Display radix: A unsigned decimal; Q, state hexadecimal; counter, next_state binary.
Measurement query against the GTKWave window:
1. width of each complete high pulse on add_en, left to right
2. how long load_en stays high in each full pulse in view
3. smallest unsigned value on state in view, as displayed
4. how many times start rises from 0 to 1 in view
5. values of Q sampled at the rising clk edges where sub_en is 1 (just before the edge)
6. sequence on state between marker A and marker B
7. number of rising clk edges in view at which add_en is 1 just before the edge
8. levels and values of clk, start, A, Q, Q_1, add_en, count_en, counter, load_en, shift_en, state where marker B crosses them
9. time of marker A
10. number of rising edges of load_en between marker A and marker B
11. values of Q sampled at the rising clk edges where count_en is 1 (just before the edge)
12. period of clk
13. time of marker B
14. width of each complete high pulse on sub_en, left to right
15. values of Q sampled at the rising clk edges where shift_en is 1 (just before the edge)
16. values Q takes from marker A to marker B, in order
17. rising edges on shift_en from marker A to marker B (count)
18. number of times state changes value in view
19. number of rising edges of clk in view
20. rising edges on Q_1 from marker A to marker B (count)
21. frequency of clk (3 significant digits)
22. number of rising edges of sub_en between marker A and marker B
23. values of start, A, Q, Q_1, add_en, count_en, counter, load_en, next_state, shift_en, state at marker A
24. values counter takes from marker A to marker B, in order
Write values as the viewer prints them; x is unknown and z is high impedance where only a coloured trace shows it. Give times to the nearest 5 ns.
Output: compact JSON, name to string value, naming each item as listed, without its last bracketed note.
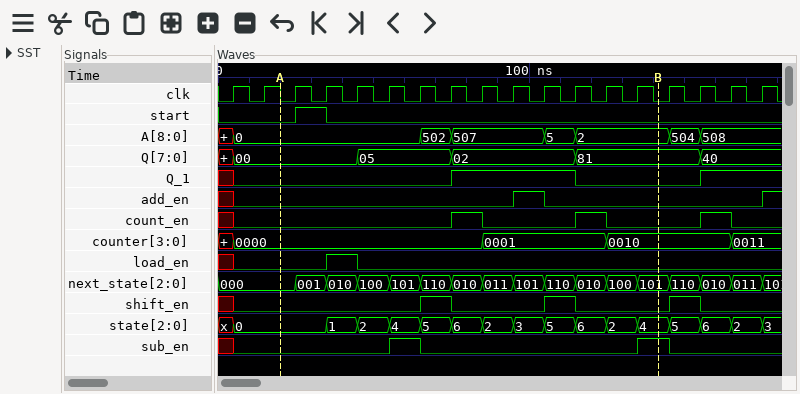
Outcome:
{"width of each complete high pulse on add_en, left to right": "10 ns", "how long load_en stays high in each full pulse in view": "10 ns", "smallest unsigned value on state in view, as displayed": "0", "how many times start rises from 0 to 1 in view": "1", "values of Q sampled at the rising clk edges where sub_en is 1": "05, 81", "sequence on state between marker A and marker B": "0, 1, 2, 4, 5, 6, 2, 3, 5, 6, 2, 4", "number of rising clk edges in view at which add_en is 1 just before the edge": "1", "levels and values of clk, start, A, Q, Q_1, add_en, count_en, counter, load_en, shift_en, state where marker B crosses them": "clk=0, start=0, A=2, Q=81, Q_1=0, add_en=0, count_en=0, counter=0010, load_en=0, shift_en=0, state=4", "time of marker A": "20 ns", "number of rising edges of load_en between marker A and marker B": "1", "values of Q sampled at the rising clk edges where count_en is 1": "02, 81, 40", "period of clk": "10 ns", "time of marker B": "140 ns", "width of each complete high pulse on sub_en, left to right": "10 ns, 10 ns", "values of Q sampled at the rising clk edges where shift_en is 1": "05, 02, 81", "values Q takes from marker A to marker B, in order": "00, 05, 02, 81", "rising edges on shift_en from marker A to marker B": "2", "number of times state changes value in view": "16", "number of rising edges of clk in view": "18", "rising edges on Q_1 from marker A to marker B": "1", "frequency of clk": "100 MHz", "number of rising edges of sub_en between marker A and marker B": "2", "values of start, A, Q, Q_1, add_en, count_en, counter, load_en, next_state, shift_en, state at marker A": "start=0, A=0, Q=00, Q_1=0, add_en=0, count_en=0, counter=0000, load_en=0, next_state=000, shift_en=0, state=0", "values counter takes from marker A to marker B, in order": "0000, 0001, 0010"}
